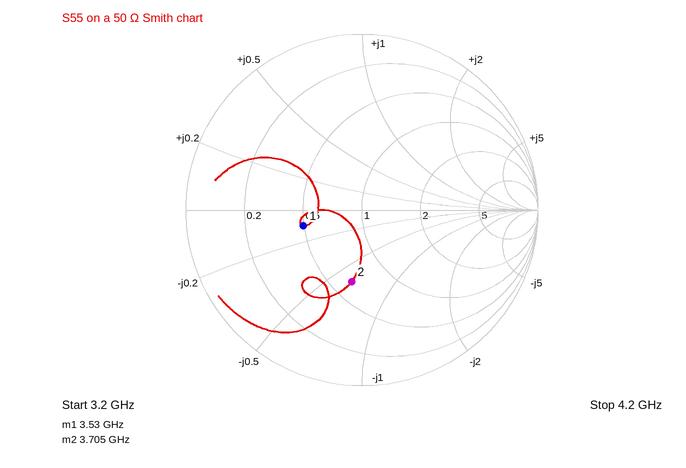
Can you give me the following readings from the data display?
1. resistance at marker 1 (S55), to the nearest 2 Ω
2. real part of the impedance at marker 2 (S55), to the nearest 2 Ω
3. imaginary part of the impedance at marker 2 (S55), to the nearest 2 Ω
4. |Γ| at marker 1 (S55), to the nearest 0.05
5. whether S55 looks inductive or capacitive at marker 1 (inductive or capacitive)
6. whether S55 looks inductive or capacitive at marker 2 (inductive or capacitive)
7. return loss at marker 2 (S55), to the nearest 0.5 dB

24 Ω
32 Ω
-32 Ω
0.35
capacitive
capacitive
7.5 dB
